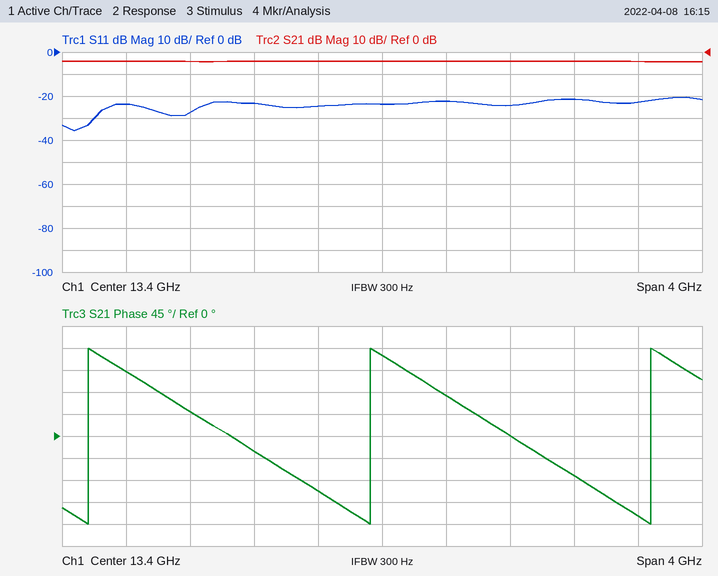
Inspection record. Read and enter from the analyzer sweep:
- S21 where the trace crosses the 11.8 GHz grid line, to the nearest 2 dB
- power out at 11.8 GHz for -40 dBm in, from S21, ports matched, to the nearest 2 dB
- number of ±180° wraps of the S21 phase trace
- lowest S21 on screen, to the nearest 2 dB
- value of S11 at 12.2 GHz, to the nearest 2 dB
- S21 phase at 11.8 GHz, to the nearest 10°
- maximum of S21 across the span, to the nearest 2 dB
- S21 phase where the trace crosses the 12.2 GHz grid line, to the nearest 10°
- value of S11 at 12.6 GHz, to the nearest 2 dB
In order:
-4 dB
-44 dBm
3
-4 dB
-28 dB
130°
-4 dB
50°
-24 dB
